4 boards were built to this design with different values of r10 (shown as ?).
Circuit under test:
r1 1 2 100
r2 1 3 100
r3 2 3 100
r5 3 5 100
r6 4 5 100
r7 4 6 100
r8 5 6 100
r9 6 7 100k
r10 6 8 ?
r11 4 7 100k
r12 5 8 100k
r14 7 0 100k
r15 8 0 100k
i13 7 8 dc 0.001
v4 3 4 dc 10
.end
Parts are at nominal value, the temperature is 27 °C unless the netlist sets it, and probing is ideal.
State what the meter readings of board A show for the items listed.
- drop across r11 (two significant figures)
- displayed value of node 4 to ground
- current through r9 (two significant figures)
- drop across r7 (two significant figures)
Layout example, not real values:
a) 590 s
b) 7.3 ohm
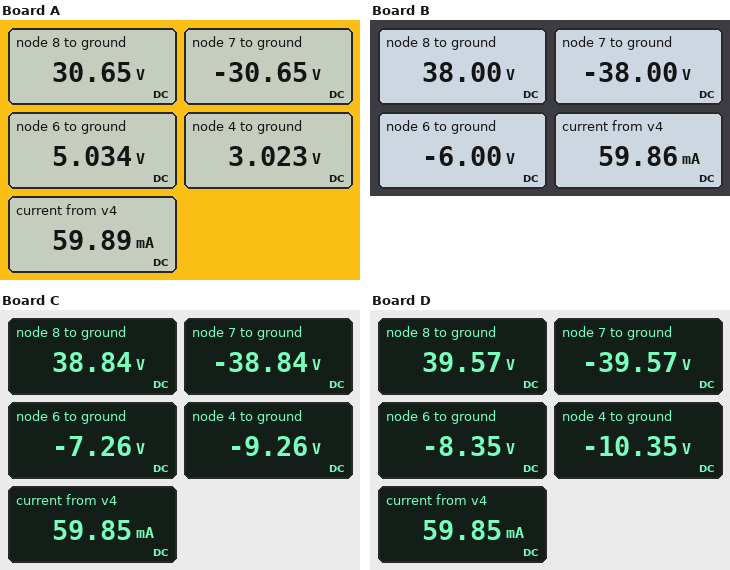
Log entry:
a) 34 V
b) 3.023 V
c) 360 µA
d) 2.0 V
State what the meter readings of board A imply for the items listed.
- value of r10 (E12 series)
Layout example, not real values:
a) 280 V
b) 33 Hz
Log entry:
a) 56 kΩ
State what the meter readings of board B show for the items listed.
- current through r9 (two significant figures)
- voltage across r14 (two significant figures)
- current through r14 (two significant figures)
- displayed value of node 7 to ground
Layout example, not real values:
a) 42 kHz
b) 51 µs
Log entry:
a) 320 µA
b) 38 V
c) 380 µA
d) -38.00 V
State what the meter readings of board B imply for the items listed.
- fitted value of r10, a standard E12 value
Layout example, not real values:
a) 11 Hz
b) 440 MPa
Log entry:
a) 220 kΩ
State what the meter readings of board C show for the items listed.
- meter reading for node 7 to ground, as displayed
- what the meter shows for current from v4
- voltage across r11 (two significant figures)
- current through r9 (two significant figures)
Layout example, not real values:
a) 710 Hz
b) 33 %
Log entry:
a) -38.84 V
b) 59.85 mA
c) 30 V
d) 320 µA
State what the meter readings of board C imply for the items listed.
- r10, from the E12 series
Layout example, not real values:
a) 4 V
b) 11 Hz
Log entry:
a) 270 kΩ
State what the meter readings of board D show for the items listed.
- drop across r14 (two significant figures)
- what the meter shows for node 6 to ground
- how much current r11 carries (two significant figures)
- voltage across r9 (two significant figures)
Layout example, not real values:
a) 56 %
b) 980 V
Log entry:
a) 40 V
b) -8.35 V
c) 290 µA
d) 31 V
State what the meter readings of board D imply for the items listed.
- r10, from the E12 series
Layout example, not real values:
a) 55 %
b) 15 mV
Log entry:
a) 330 kΩ
